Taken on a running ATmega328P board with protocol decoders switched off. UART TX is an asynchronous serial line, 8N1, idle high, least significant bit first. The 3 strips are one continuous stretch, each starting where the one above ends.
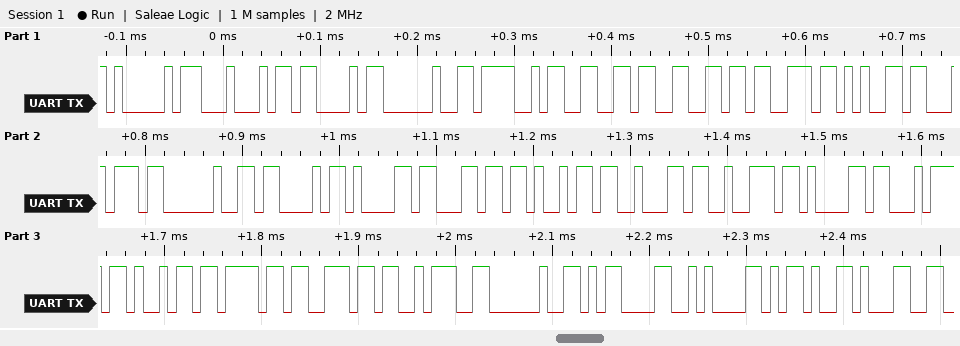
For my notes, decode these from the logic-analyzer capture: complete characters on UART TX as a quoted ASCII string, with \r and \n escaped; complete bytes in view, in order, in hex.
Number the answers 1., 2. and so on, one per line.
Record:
1. "ADC Offset Calibration: \r\n-1"
2. 41 44 43 20 4F 66 66 73 65 74 20 43 61 6C 69 62 72 61 74 69 6F 6E 3A 20 0D 0A 2D 31
